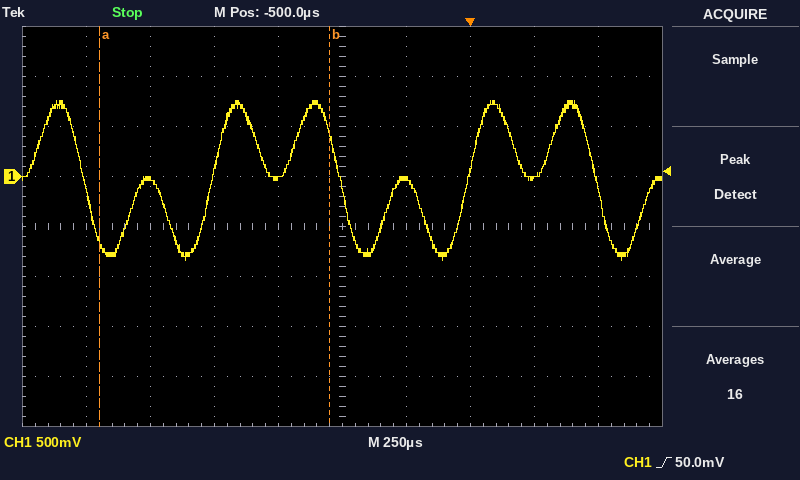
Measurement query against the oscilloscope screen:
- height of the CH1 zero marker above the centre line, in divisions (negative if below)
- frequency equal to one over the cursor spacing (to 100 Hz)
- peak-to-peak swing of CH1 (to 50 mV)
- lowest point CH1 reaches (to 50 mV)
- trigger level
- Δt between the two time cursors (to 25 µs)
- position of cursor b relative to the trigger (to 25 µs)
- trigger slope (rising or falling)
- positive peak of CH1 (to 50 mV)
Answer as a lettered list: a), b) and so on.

a) +1.0 div
b) 1.1 kHz
c) 1.60 V
d) -850 mV
e) 50.0 mV
f) 900 µs
g) -550 µs
h) rising
i) 750 mV
